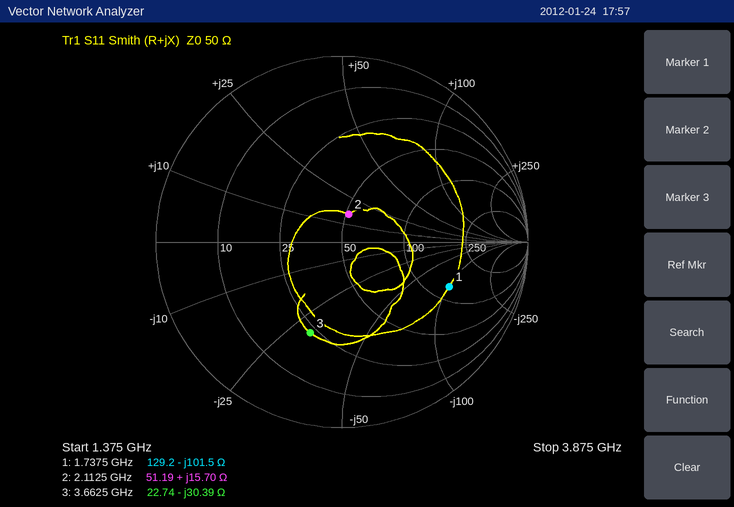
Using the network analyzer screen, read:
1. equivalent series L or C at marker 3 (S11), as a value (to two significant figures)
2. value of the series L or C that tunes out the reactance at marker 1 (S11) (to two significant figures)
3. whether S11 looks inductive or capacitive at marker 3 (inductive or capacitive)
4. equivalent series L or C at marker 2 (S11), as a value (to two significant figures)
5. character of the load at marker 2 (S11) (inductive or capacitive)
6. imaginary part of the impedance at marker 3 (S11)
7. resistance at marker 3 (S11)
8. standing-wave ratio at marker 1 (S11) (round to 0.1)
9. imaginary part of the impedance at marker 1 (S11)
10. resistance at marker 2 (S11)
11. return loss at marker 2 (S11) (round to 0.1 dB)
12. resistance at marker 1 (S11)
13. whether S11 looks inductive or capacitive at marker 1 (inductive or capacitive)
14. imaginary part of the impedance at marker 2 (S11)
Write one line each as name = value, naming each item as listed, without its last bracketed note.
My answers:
equivalent series L or C at marker 3 (S11), as a value = 1.4 pF
value of the series L or C that tunes out the reactance at marker 1 (S11) = 9.3 nH
whether S11 looks inductive or capacitive at marker 3 = capacitive
equivalent series L or C at marker 2 (S11), as a value = 1.2 nH
character of the load at marker 2 (S11) = inductive
imaginary part of the impedance at marker 3 = -30.39 Ω
resistance at marker 3 = 22.74 Ω
standing-wave ratio at marker 1 (S11) = 4.3
imaginary part of the impedance at marker 1 = -101.5 Ω
resistance at marker 2 = 51.19 Ω
return loss at marker 2 (S11) = 16.3 dB
resistance at marker 1 = 129.2 Ω
whether S11 looks inductive or capacitive at marker 1 = capacitive
imaginary part of the impedance at marker 2 = +15.70 Ω
